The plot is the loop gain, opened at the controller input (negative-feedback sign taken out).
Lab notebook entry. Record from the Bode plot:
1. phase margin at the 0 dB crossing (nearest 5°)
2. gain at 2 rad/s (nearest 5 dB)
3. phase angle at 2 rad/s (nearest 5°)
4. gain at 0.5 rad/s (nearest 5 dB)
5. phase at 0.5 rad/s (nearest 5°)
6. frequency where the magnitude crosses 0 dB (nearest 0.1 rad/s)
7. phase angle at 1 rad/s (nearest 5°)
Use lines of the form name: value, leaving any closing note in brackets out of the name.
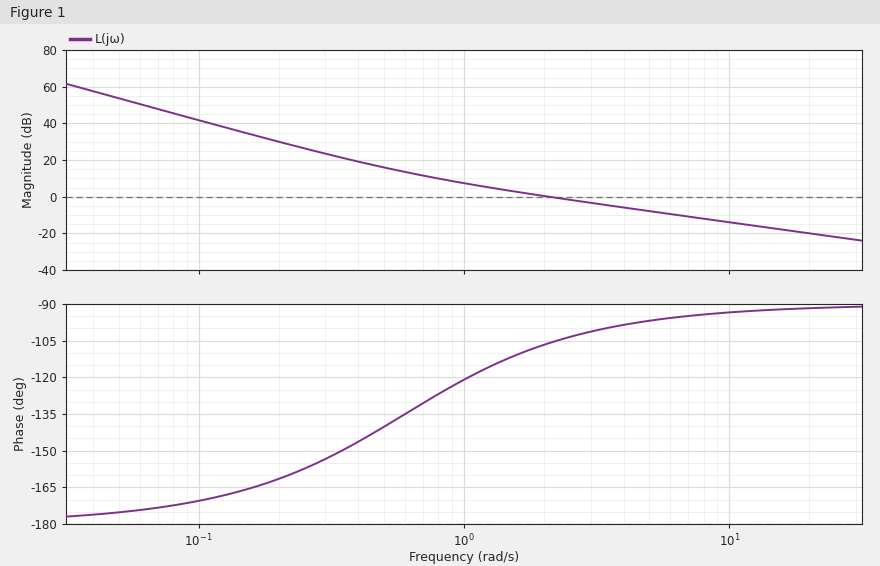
phase margin at the 0 dB crossing: 75°
gain at 2 rad/s: 0 dB
phase angle at 2 rad/s: -105°
gain at 0.5 rad/s: 15 dB
phase at 0.5 rad/s: -140°
frequency where the magnitude crosses 0 dB: 2.1 rad/s
phase angle at 1 rad/s: -120°
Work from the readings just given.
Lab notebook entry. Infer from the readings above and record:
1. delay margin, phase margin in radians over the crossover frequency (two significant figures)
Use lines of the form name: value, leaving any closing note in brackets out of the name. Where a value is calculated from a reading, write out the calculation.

delay margin, phase margin in radians over the crossover frequency: 75 × π / 180 / 2.1 = 0.62 s
